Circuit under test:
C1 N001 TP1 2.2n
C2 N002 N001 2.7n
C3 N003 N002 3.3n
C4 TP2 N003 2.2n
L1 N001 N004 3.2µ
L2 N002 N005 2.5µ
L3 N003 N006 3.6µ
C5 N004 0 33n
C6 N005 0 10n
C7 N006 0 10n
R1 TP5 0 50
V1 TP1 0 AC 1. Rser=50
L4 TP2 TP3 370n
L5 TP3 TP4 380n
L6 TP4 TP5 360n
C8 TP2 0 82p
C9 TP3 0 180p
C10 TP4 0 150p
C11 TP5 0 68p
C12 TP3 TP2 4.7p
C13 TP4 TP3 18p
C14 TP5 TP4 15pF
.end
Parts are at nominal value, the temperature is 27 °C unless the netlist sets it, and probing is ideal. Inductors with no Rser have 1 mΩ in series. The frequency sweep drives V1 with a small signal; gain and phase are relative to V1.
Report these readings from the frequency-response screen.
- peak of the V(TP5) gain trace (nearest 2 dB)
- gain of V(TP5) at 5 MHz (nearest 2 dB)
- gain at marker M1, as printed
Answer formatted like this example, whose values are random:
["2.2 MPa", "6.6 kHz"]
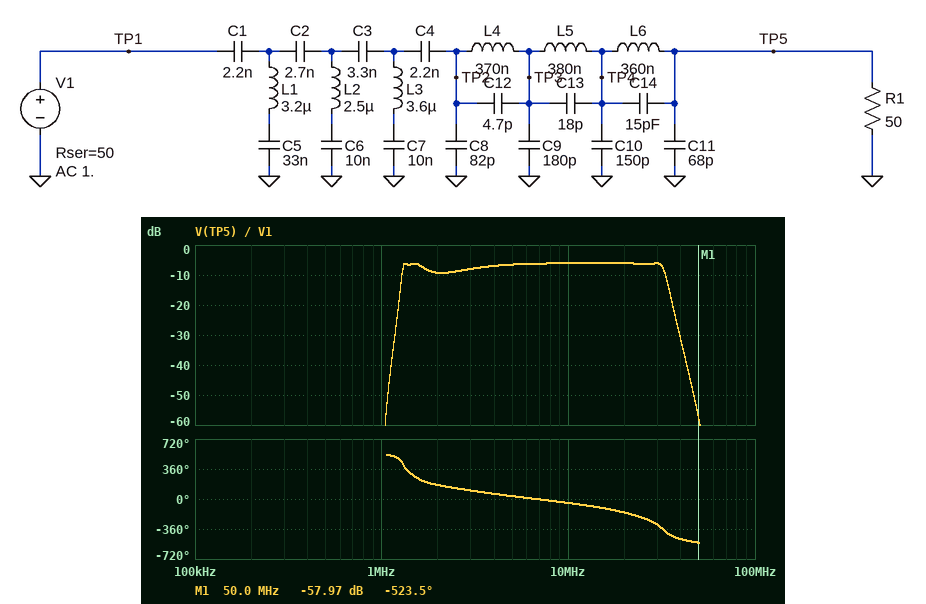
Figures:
["-6 dB", "-6 dB", "-57.97 dB"]
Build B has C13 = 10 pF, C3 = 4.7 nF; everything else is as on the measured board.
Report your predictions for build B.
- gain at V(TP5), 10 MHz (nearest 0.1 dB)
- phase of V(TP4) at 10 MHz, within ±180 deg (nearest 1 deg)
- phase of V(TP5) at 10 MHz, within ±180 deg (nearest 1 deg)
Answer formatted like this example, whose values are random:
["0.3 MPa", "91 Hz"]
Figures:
["-6.1 dB", "-21 deg", "-48 deg"]
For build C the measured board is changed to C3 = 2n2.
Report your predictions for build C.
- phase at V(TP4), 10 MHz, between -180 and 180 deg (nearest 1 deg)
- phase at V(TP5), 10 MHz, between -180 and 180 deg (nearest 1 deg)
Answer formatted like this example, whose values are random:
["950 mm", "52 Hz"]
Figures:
["-19 deg", "-46 deg"]
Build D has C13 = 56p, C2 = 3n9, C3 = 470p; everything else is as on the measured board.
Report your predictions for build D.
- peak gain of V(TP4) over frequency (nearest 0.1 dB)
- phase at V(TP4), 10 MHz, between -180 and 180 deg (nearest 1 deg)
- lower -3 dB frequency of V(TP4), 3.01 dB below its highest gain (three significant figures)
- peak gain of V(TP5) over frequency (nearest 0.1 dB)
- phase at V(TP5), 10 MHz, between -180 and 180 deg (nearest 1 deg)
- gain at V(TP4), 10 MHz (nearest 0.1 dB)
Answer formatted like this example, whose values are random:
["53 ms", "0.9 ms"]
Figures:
["-4.5 dB", "-5 deg", "4.26 MHz", "-6.2 dB", "-32 deg", "-6.1 dB"]
